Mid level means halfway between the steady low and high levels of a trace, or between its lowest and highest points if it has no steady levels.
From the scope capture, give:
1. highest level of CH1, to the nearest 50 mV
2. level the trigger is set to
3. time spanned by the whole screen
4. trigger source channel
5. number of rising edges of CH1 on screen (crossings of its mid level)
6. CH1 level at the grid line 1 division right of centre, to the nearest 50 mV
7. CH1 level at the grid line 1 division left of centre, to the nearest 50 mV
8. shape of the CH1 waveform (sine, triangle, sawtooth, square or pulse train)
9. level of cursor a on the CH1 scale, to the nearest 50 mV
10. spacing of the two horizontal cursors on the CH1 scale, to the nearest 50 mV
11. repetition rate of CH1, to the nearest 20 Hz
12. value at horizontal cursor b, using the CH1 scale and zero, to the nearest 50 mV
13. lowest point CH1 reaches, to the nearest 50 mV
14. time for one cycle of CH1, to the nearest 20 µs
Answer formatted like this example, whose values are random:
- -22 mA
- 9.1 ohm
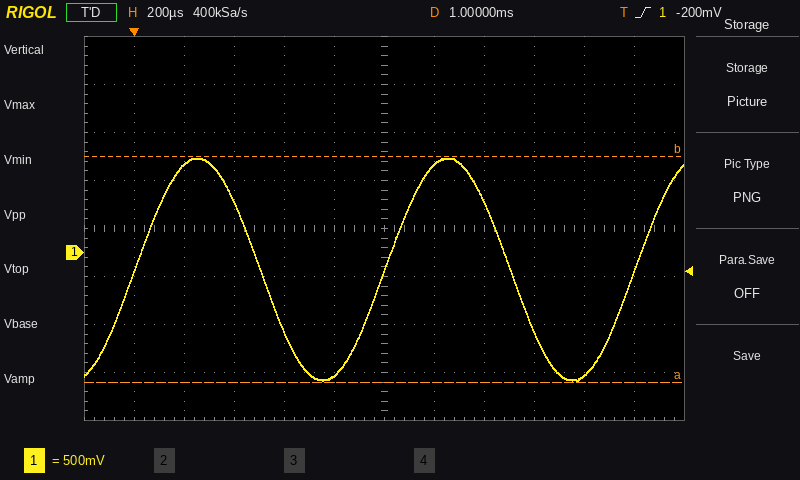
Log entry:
- 1.00 V
- -200 mV
- 2.4 ms
- CH1
- 3
- 900 mV
- -1.30 V
- sine
- -1.35 V
- 2.35 V
- 1.00 kHz
- 1.00 V
- -1.35 V
- 1.00 ms
